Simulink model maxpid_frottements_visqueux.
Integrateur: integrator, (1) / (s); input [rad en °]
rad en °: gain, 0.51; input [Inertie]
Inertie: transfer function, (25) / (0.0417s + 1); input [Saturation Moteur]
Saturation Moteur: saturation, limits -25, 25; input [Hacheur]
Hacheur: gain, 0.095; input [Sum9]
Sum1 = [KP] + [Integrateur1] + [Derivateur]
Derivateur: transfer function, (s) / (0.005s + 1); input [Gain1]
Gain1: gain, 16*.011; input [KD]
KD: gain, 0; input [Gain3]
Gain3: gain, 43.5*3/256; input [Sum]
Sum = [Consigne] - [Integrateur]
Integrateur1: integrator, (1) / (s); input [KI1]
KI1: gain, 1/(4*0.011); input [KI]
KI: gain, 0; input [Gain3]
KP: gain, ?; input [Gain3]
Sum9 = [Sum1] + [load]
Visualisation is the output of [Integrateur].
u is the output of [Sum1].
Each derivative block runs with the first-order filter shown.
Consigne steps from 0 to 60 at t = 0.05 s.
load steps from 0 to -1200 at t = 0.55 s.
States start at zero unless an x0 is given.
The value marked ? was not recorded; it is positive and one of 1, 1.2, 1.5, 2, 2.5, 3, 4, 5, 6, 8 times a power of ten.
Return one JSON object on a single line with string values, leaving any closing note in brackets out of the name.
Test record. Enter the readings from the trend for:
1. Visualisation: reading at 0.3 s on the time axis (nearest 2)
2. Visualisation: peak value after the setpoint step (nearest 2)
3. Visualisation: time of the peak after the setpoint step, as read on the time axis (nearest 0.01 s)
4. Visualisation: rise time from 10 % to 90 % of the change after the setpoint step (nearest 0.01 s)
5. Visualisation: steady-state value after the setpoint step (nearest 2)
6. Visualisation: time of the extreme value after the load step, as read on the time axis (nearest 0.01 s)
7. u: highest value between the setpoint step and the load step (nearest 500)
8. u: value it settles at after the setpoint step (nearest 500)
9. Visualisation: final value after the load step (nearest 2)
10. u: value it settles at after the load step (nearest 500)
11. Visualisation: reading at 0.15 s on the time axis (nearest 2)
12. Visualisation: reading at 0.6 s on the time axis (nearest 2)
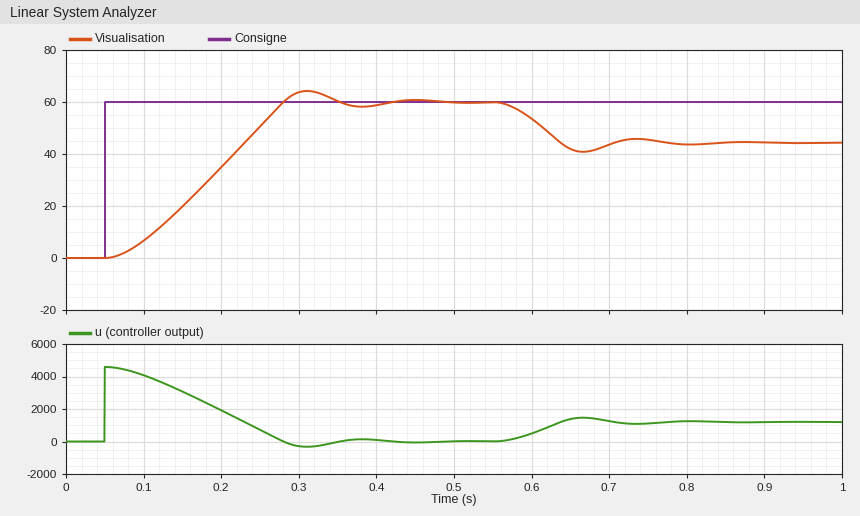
{"Visualisation: reading at 0.3 s on the time axis": "64", "Visualisation: peak value after the setpoint step": "64", "Visualisation: time of the peak after the setpoint step, as read on the time axis": "0.31 s", "Visualisation: rise time from 10 % to 90 % of the change after the setpoint step": "0.16 s", "Visualisation: steady-state value after the setpoint step": "60", "Visualisation: time of the extreme value after the load step, as read on the time axis": "0.67 s", "u: highest value between the setpoint step and the load step": "4500", "u: value it settles at after the setpoint step": "0", "Visualisation: final value after the load step": "44", "u: value it settles at after the load step": "1000", "Visualisation: reading at 0.15 s on the time axis": "20", "Visualisation: reading at 0.6 s on the time axis": "54"}
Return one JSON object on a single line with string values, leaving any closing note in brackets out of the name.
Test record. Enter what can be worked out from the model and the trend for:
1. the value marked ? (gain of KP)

{"the value marked ?": "150"}
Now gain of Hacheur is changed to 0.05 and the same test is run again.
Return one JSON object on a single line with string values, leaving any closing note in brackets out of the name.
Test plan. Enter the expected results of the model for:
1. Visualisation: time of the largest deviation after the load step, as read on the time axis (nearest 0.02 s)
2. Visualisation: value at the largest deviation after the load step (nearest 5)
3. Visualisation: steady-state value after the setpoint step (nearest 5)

{"Visualisation: time of the largest deviation after the load step, as read on the time axis": "0.68 s", "Visualisation: value at the largest deviation after the load step": "40", "Visualisation: steady-state value after the setpoint step": "60"}
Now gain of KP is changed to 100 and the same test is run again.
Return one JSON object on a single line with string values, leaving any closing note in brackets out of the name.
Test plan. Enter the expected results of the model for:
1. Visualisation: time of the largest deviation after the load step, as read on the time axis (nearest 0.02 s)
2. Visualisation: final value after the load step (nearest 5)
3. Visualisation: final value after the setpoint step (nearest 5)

{"Visualisation: time of the largest deviation after the load step, as read on the time axis": "0.70 s", "Visualisation: final value after the load step": "35", "Visualisation: final value after the setpoint step": "60"}
